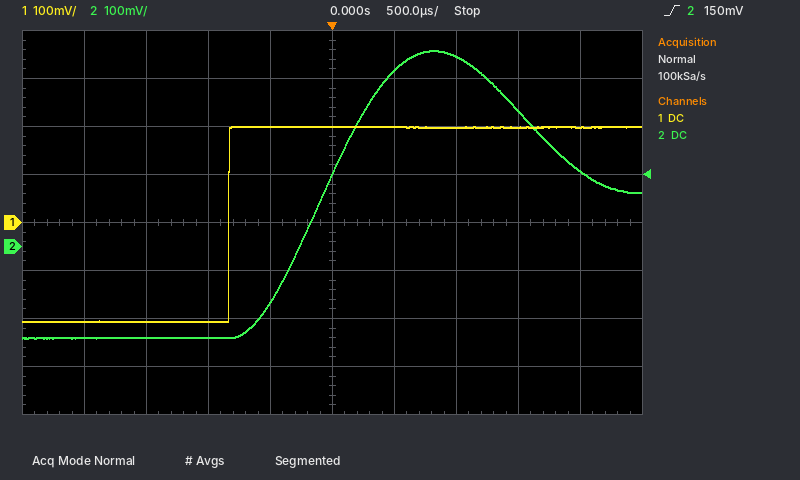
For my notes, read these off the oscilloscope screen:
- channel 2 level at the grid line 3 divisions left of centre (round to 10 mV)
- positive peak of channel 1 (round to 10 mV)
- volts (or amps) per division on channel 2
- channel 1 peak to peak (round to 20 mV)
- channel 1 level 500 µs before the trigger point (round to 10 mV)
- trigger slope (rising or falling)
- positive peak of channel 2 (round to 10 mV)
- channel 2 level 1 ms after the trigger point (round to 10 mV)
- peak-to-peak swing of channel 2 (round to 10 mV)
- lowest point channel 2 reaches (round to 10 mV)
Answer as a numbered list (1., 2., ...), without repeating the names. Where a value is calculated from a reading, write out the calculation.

1. -190 mV
2. 200 mV
3. 100 mV
4. 400 mV
5. 200 mV
6. rising
7. 410 mV
8. 400 mV
9. 410 mV − (-190 mV) = 600 mV
10. -190 mV
